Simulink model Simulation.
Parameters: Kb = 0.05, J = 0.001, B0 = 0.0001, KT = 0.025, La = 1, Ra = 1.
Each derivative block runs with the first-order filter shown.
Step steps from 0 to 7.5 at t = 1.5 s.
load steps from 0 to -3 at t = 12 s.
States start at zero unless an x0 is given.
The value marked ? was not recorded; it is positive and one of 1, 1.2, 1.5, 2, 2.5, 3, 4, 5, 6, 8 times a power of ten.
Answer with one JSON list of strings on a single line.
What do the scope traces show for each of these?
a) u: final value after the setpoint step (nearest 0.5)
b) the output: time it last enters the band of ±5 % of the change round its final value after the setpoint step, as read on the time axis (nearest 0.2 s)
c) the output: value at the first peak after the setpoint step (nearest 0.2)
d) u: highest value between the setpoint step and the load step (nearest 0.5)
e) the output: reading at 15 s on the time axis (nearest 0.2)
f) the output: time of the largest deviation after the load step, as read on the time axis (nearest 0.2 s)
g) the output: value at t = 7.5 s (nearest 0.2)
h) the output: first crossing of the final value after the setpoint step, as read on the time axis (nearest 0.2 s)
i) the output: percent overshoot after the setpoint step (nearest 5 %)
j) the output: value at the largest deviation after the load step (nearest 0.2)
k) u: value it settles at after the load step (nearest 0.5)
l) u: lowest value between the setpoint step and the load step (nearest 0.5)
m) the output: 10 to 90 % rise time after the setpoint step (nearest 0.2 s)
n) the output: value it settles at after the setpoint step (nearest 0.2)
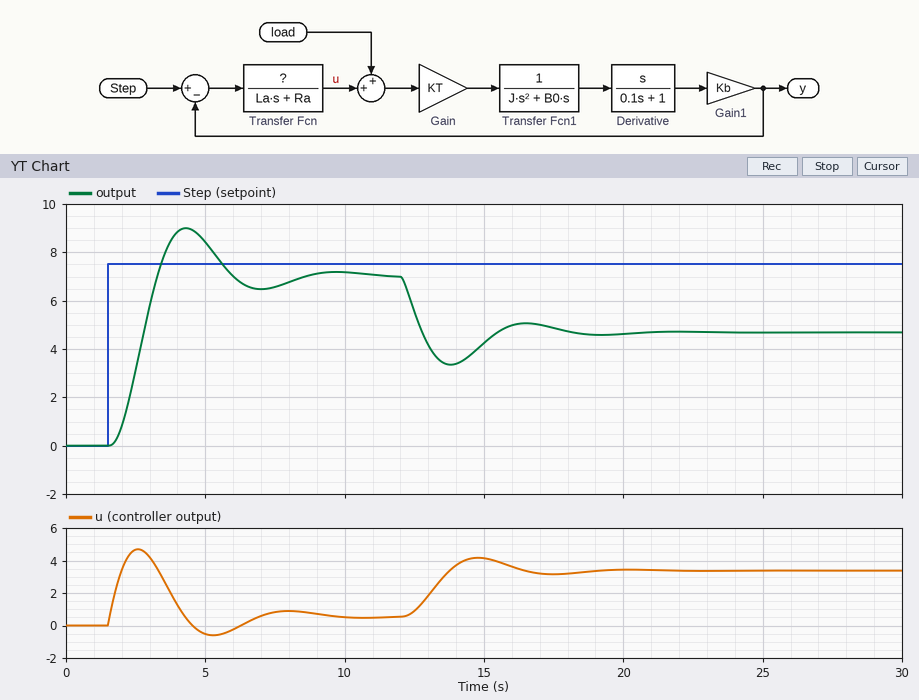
["0.5", "7.8 s", "9.0", "4.5", "4.2", "13.8 s", "6.6", "3.2 s", "30 %", "3.4", "3.5", "-0.5", "1.2 s", "7.0"]
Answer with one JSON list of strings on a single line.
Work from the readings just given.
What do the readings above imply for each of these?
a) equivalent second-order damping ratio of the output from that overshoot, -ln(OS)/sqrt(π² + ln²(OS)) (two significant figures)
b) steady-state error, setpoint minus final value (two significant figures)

["0.36", "0.50"]
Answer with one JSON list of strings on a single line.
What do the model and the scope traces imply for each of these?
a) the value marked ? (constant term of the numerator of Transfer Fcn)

["1.2"]
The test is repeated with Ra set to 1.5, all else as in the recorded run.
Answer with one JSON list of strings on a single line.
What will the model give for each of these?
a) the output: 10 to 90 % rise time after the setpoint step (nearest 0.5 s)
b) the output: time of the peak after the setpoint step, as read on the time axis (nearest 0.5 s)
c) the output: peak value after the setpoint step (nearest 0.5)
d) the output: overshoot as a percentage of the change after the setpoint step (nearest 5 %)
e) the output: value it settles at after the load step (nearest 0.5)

["1.5 s", "4.5 s", "7.5", "10 %", "3.5"]
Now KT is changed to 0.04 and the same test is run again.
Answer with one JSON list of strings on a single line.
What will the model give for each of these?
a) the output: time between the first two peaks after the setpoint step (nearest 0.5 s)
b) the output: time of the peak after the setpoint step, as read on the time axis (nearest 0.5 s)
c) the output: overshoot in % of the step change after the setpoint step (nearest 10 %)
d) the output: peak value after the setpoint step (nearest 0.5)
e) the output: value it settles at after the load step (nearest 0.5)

["4.0 s", "3.5 s", "40 %", "10.0", "5.0"]
